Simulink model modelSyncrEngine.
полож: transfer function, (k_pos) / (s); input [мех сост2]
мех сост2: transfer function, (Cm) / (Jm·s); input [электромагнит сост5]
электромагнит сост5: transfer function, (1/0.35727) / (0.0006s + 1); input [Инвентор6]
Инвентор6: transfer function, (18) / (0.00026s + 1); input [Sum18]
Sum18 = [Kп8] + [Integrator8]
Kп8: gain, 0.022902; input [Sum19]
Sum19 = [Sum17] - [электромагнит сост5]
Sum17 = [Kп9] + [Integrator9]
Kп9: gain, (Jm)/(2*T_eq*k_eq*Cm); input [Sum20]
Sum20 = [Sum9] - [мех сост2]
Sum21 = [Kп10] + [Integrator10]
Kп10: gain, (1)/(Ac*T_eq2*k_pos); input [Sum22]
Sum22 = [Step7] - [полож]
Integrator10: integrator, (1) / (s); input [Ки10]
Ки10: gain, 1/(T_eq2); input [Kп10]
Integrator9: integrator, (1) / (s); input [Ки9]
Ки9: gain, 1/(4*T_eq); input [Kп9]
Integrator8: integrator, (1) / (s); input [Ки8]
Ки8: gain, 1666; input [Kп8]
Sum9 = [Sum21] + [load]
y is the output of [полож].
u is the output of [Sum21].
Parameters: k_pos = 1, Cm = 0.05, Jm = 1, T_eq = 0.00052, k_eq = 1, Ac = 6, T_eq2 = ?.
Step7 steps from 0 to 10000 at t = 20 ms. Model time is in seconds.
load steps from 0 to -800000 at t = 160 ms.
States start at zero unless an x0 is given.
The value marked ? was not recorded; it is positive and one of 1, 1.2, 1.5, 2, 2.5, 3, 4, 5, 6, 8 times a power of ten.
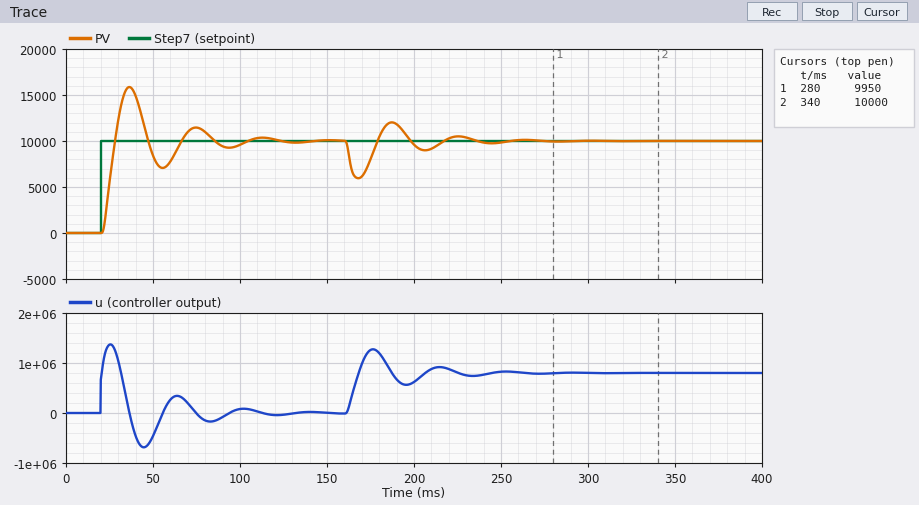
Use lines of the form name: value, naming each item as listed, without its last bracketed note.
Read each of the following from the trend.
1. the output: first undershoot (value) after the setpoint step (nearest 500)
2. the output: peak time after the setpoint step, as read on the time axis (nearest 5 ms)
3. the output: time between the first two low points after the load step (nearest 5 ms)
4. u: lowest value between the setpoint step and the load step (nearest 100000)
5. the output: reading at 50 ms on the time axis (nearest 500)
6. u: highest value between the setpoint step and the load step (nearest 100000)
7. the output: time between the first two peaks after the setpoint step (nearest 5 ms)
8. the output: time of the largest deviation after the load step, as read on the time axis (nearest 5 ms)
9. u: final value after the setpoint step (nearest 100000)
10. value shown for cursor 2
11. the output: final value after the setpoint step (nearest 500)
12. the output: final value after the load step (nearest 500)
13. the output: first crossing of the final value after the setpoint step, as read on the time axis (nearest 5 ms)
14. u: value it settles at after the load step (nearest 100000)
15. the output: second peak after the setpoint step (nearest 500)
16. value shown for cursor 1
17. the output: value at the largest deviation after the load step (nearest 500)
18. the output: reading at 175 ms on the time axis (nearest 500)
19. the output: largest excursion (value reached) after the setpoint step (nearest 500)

the output: first undershoot (value) after the setpoint step: 7000
the output: peak time after the setpoint step, as read on the time axis: 35 ms
the output: time between the first two low points after the load step: 40 ms
u: lowest value between the setpoint step and the load step: -700000
the output: reading at 50 ms on the time axis: 8500
u: highest value between the setpoint step and the load step: 1400000
the output: time between the first two peaks after the setpoint step: 40 ms
the output: time of the largest deviation after the load step, as read on the time axis: 170 ms
u: final value after the setpoint step: 0
value shown for cursor 2: 10000
the output: final value after the setpoint step: 10000
the output: final value after the load step: 10000
the output: first crossing of the final value after the setpoint step, as read on the time axis: 30 ms
u: value it settles at after the load step: 800000
the output: second peak after the setpoint step: 11500
value shown for cursor 1: 9950
the output: value at the largest deviation after the load step: 6000
the output: reading at 175 ms on the time axis: 8000
the output: largest excursion (value reached) after the setpoint step: 16000
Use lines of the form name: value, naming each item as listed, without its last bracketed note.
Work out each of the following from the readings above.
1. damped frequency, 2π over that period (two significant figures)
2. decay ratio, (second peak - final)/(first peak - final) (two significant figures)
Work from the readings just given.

damped frequency, 2π over that period: 0.16 rad/ms
decay ratio, (second peak - final)/(first peak - final): 0.25
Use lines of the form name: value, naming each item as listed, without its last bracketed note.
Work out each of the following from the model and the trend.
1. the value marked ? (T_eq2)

the value marked ?: 0.0025
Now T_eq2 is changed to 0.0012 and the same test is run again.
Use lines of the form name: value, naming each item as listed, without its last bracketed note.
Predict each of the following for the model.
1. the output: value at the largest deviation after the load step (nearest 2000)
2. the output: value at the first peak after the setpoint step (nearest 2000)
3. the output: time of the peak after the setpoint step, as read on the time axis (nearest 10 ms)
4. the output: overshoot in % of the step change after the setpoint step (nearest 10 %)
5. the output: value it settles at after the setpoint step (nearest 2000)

the output: value at the largest deviation after the load step: 8000
the output: value at the first peak after the setpoint step: 18000
the output: time of the peak after the setpoint step, as read on the time axis: 30 ms
the output: overshoot in % of the step change after the setpoint step: 80 %
the output: value it settles at after the setpoint step: 10000
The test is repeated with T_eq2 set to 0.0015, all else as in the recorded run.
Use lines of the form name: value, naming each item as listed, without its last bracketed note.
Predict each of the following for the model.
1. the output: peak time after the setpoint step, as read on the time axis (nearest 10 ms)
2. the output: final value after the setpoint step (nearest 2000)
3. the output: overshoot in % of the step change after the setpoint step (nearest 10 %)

the output: peak time after the setpoint step, as read on the time axis: 30 ms
the output: final value after the setpoint step: 10000
the output: overshoot in % of the step change after the setpoint step: 70 %
